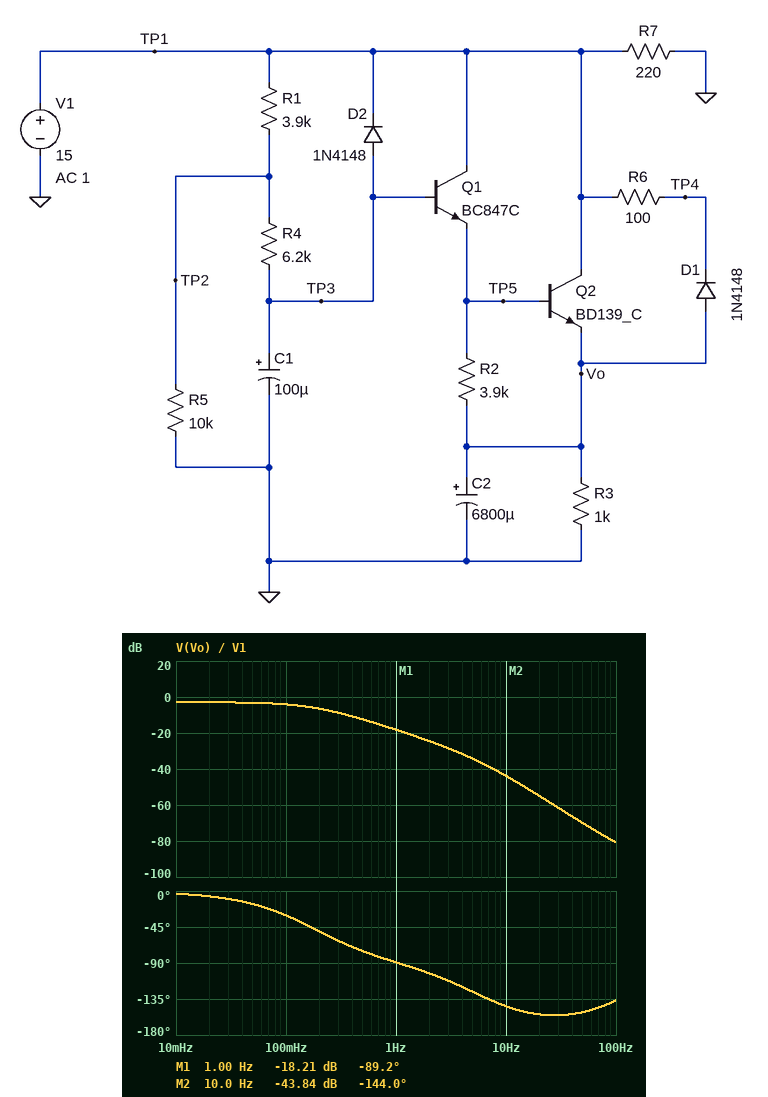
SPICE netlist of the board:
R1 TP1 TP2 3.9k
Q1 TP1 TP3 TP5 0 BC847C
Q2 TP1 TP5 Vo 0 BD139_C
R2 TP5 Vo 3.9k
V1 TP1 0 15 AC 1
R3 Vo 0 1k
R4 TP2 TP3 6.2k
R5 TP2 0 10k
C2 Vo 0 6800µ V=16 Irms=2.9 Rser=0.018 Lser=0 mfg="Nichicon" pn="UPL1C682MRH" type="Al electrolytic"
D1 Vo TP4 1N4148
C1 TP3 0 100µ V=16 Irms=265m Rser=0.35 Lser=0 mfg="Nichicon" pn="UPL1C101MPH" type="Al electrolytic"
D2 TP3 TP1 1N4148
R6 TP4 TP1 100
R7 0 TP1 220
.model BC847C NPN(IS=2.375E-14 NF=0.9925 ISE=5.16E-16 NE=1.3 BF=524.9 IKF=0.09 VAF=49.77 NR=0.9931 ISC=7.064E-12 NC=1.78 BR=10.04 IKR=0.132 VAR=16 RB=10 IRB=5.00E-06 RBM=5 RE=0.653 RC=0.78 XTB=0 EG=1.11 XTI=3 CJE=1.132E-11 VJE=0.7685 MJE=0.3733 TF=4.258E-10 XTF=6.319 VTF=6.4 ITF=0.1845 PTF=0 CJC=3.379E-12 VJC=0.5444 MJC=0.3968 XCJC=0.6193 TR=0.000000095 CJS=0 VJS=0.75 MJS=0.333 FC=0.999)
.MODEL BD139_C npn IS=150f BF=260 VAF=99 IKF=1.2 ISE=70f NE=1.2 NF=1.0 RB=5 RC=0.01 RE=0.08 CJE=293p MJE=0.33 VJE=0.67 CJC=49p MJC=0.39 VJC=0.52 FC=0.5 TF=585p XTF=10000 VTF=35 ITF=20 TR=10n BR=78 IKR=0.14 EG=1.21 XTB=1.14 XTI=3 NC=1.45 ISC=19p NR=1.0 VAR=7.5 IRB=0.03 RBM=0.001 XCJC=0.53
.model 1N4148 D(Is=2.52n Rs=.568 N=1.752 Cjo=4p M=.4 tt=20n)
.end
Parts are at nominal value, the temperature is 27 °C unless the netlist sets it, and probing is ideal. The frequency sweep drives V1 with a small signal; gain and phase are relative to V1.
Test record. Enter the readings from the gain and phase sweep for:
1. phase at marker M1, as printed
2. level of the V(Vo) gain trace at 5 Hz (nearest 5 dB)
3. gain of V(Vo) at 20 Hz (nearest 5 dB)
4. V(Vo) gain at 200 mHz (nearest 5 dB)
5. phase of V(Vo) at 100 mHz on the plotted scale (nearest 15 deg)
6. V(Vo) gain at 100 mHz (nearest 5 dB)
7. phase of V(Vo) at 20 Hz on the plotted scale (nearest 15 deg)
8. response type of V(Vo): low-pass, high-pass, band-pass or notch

-89.2 deg
-35 dB
-55 dB
-5 dB
-30 deg
-5 dB
-150 deg
low-pass
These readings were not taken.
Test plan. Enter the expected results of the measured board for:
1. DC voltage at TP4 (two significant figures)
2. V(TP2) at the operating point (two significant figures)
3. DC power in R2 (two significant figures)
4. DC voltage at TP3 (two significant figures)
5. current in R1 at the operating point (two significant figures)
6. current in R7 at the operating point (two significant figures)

15 V
11 V
110 µW
11 V
1.1 mA
68 mA
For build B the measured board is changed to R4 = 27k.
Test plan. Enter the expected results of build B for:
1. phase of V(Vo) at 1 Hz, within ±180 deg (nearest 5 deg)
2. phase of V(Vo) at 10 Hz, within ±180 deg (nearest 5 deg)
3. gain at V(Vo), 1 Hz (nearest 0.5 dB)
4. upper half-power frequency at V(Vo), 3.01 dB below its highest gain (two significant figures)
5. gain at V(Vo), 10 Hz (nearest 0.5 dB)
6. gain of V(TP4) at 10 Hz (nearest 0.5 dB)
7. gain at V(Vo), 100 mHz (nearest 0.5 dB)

-95 deg
-135 deg
-28.5 dB
53 mHz
-54.0 dB
0 dB
-9.5 dB
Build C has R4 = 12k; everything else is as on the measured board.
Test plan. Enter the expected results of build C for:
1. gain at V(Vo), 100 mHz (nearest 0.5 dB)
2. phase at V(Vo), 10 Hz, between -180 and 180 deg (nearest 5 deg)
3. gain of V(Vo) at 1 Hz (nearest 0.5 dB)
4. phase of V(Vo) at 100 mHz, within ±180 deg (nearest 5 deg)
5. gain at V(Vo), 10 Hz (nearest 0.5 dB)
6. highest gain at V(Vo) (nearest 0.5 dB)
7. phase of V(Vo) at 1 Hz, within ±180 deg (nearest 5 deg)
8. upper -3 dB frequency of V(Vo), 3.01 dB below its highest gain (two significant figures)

-5.5 dB
-140 deg
-22.5 dB
-45 deg
-48.0 dB
-3.0 dB
-95 deg
110 mHz
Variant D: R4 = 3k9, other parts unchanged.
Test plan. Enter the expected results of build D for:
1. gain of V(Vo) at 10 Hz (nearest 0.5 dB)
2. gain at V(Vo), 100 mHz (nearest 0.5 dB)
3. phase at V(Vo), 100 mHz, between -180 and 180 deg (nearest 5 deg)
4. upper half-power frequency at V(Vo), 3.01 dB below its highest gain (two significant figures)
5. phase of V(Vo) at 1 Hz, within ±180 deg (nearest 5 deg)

-41.5 dB
-3.5 dB
-25 deg
240 mHz
-85 deg
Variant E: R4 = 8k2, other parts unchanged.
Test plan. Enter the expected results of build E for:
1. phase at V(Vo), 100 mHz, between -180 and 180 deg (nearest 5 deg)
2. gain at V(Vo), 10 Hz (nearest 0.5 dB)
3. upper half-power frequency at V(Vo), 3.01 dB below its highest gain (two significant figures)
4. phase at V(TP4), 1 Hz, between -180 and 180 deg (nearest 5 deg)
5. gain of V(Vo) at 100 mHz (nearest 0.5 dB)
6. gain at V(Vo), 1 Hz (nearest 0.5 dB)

-35 deg
-45.5 dB
140 mHz
0 deg
-4.5 dB
-20.0 dB
